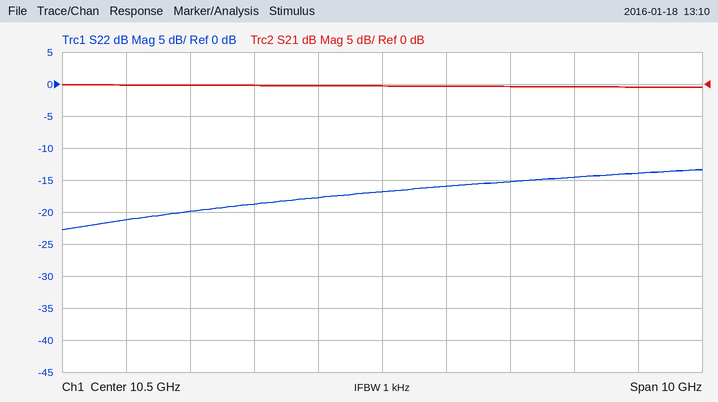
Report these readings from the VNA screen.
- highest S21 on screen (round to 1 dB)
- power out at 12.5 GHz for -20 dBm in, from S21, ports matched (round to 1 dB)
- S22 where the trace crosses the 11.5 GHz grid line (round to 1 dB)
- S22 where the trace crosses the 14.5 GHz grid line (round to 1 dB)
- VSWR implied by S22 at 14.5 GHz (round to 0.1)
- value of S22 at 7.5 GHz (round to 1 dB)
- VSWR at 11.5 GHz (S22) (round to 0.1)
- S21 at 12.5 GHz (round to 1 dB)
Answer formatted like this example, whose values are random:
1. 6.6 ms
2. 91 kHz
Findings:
1. 0 dB
2. -20 dBm
3. -16 dB
4. -14 dB
5. 1.5
6. -20 dB
7. 1.4
8. 0 dB
